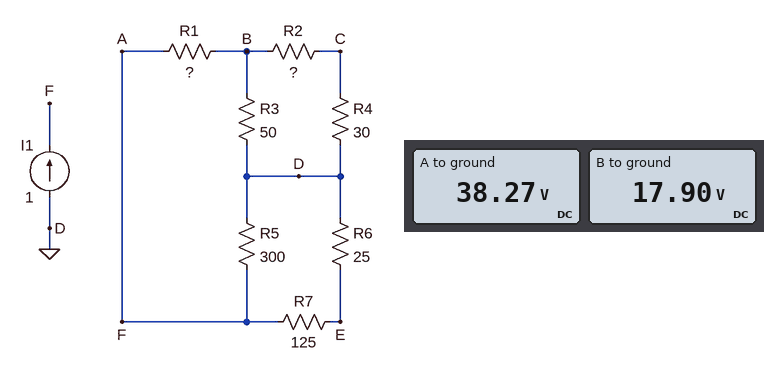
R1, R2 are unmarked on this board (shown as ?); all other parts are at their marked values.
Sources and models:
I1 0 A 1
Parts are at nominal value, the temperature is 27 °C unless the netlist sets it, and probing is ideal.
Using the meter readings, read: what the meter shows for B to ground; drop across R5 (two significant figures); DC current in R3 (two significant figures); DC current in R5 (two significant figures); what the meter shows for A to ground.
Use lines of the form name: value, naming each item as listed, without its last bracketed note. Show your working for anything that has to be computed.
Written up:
what the meter shows for B to ground: 17.90 V
drop across R5: 38.27 V = 38 V
DC current in R3: (17.9 V) / 50 Ω = 360 mA
DC current in R5: (38.27 V) / 300 Ω = 130 mA
what the meter shows for A to ground: 38.27 V
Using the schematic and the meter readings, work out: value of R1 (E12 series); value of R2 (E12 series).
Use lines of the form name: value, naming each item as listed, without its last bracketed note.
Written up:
value of R1: 33 Ω
value of R2: 39 Ω
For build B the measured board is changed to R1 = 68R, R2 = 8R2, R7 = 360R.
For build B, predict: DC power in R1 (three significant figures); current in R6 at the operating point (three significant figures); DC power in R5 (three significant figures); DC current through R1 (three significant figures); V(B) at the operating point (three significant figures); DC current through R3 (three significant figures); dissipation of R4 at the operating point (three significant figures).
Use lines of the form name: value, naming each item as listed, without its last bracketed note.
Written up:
DC power in R1: 29.0 W
current in R6 at the operating point: 152 mA
DC power in R5: 11.4 W
DC current through R1: 653 mA
V(B) at the operating point: 14.1 V
DC current through R3: 283 mA
dissipation of R4 at the operating point: 4.11 W
